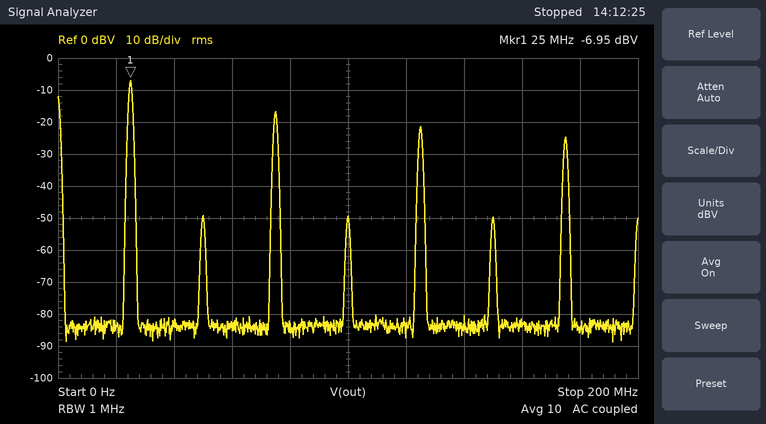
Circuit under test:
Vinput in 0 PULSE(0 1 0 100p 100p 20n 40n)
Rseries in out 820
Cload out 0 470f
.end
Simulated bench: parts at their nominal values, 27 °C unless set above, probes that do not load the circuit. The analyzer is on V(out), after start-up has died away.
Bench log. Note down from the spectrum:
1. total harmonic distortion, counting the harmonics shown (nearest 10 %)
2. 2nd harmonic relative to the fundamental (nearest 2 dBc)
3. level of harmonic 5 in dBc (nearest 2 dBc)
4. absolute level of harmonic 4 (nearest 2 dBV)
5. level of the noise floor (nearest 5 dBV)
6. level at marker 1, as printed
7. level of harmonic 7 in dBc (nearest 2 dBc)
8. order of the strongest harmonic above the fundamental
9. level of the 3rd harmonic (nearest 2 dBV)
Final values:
40 %
-42 dBc
-14 dBc
-50 dBV
-85 dBV
-6.95 dBV
-18 dBc
3
-16 dBV
